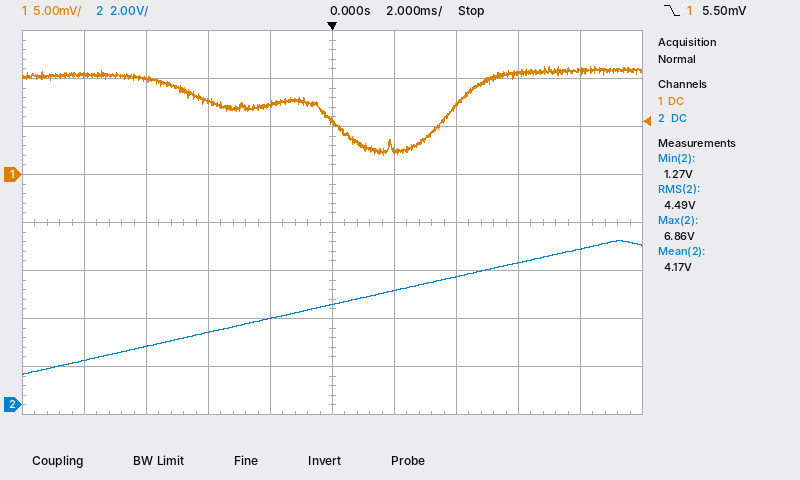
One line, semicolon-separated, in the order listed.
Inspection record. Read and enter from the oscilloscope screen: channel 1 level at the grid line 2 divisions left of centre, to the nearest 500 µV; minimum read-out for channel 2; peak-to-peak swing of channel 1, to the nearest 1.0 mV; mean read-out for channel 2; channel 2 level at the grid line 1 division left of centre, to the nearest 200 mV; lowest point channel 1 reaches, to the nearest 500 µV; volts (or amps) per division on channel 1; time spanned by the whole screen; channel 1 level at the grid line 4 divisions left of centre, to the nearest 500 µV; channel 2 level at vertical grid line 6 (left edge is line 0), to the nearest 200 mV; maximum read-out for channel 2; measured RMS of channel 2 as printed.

7.5 mV; 1.27 V; 9.0 mV; 4.17 V; 3.6 V; 2.0 mV; 5 mV; 20 ms; 10.5 mV; 4.8 V; 6.86 V; 4.49 V
